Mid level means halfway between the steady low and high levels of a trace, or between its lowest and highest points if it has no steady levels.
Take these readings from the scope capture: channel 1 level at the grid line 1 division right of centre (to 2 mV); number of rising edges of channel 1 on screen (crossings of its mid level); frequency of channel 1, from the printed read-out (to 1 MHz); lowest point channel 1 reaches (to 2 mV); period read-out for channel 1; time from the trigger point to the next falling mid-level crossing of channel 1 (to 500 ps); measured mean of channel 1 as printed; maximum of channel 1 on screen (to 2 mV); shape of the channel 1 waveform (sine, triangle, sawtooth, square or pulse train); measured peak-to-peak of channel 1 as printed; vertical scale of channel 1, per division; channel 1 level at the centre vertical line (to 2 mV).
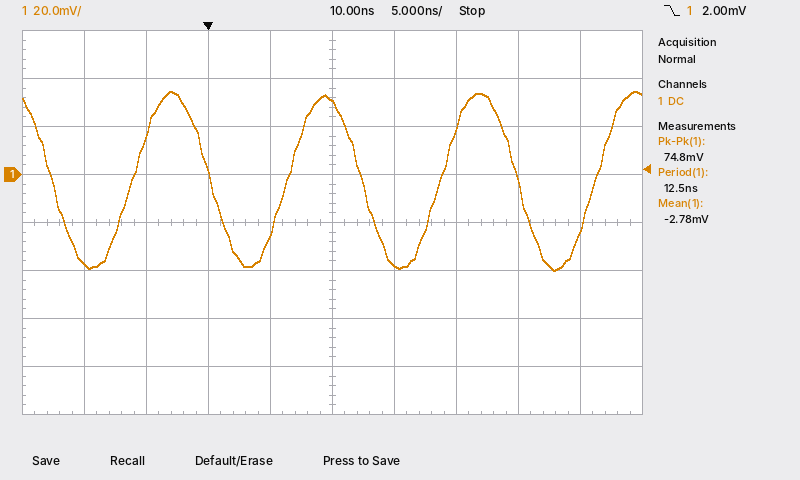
-38 mV
4
80 MHz
-40 mV
12.5 ns
12.5 ns
-2.78 mV
34 mV
sine
74.8 mV
20 mV
30 mV
